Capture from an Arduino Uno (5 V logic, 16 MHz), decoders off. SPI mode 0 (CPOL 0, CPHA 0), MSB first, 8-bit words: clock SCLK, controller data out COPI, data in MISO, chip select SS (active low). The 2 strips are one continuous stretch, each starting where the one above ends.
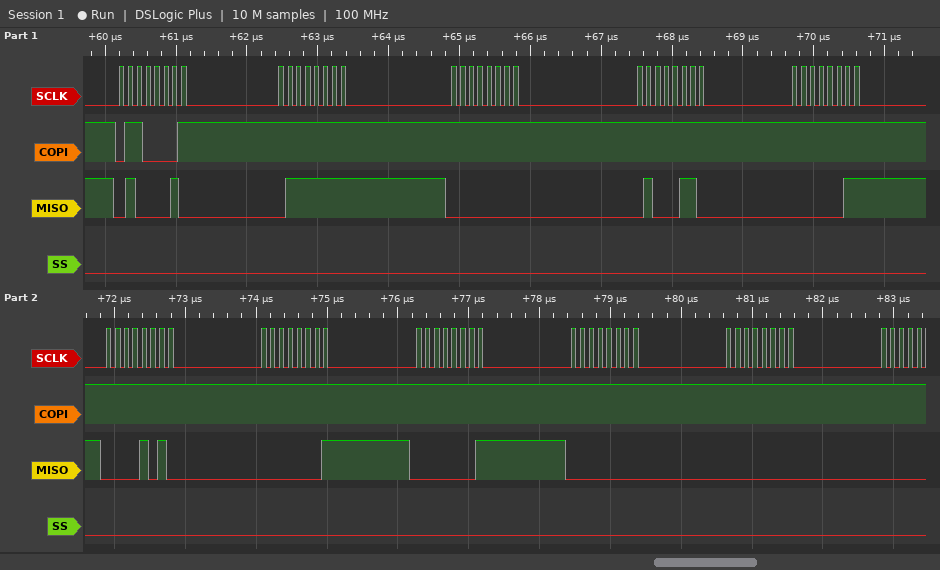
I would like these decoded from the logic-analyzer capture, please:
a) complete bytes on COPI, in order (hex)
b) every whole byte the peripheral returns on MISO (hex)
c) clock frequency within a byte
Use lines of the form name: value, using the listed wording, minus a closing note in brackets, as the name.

complete bytes on COPI, in order: 61 FF FF FF FF FF FF FF FF FF
every whole byte the peripheral returns on MISO: 42 7F 00 46 03 0A 01 01 00 00
clock frequency within a byte: 8 MHz
